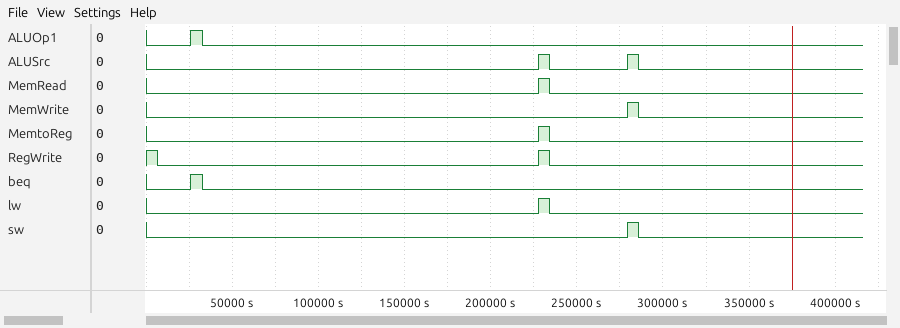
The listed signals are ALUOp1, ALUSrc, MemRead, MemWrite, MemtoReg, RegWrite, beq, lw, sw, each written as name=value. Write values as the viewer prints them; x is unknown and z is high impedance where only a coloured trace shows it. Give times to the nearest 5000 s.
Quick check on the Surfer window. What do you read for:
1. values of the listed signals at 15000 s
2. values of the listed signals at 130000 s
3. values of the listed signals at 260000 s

ALUOp1=0, ALUSrc=0, MemRead=0, MemWrite=0, MemtoReg=0, RegWrite=0, beq=0, lw=0, sw=0
ALUOp1=0, ALUSrc=0, MemRead=0, MemWrite=0, MemtoReg=0, RegWrite=0, beq=0, lw=0, sw=0
ALUOp1=0, ALUSrc=0, MemRead=0, MemWrite=0, MemtoReg=0, RegWrite=0, beq=0, lw=0, sw=0
